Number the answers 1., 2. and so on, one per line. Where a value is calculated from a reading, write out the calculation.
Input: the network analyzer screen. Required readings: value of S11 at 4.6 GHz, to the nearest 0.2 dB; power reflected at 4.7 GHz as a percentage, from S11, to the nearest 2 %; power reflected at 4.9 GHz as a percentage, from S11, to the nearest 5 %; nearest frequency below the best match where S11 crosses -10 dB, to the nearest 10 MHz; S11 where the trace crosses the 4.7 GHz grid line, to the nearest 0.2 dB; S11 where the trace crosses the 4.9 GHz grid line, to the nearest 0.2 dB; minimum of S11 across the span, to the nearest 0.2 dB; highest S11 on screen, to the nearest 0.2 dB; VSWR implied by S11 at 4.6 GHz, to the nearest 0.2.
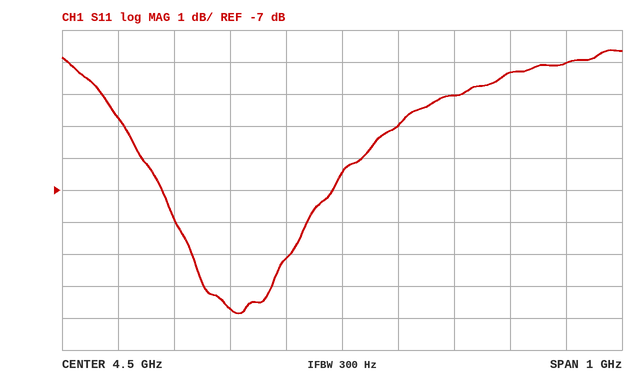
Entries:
1. -5.0 dB
2. 10^(-4/10) ≈ 40 %
3. 10^(-3/10) ≈ 50 %
4. 4.25 GHz
5. -4.0 dB
6. -3.0 dB
7. -10.8 dB
8. -2.6 dB
9. |Γ| = 10^(-5/20) = 0.5623; VSWR = (1 + 0.5623)/(1 − 0.5623) ≈ 3.6
